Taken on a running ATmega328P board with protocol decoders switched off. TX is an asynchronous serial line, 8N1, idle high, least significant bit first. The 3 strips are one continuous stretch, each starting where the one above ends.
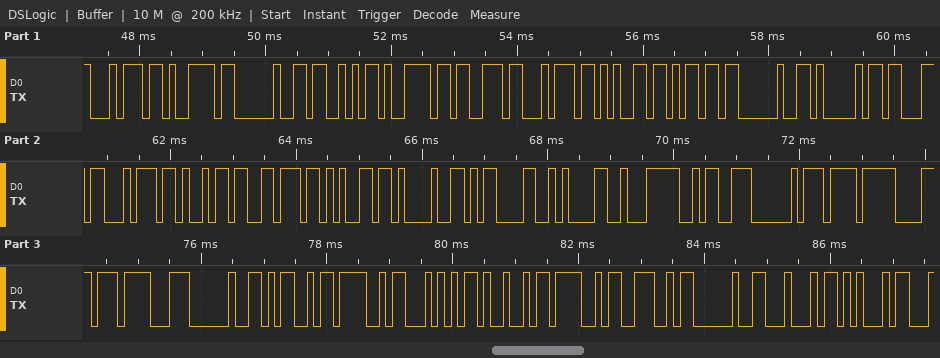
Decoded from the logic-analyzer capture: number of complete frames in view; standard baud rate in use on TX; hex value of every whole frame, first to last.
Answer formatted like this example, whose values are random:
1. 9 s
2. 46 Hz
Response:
1. 35
2. 9600 baud
3. 74 79 20 53 79 73 74 65 6D 20 41 63 74 69 76 65 21 0D 0A E2 9A A0 EF B8 8F 20 4D 4F 54 49 4F 4E 20 44 45
